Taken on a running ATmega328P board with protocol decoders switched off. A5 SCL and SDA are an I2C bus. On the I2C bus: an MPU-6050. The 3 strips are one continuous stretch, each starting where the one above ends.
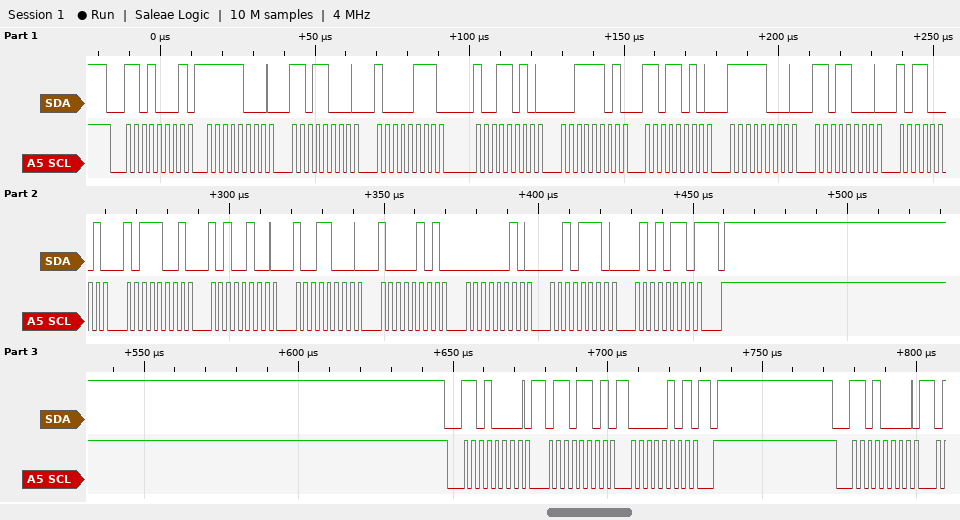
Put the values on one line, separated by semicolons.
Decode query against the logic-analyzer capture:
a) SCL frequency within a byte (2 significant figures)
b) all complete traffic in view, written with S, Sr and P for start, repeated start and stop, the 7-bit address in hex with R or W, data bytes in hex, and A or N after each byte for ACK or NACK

400 kHz; S 68R A F8 A D8 A 87 A 9A A 3D A DA A F8 A D8 A B1 A B9 A A4 A 98 A 85 A 02 A 2E A 56 N P S 68W A 6D A 05 A P S 68W A
